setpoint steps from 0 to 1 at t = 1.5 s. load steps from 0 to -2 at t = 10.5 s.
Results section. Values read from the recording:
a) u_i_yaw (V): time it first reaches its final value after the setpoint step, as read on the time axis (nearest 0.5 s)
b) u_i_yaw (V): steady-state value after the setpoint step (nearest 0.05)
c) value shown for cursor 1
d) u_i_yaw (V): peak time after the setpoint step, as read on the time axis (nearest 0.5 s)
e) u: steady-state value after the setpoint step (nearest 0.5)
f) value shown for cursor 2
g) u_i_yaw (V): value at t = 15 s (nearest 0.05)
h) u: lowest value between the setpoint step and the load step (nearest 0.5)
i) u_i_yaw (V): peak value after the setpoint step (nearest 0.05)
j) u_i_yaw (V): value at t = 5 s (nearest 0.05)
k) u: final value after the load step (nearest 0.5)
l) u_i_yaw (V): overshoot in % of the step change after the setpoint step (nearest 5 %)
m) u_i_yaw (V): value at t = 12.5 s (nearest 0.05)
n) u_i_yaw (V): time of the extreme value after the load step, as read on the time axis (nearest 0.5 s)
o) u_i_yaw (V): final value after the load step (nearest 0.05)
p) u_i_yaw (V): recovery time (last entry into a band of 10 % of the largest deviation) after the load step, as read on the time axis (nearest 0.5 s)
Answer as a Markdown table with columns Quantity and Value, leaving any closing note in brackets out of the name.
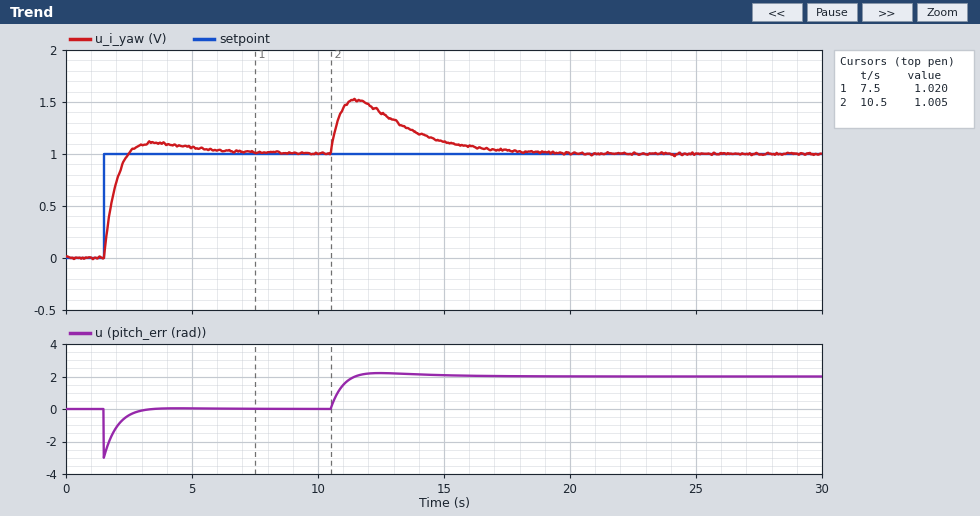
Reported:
| Quantity | Value |
|---|---|
| u_i_yaw (V): time it first reaches its final value after the setpoint step, as read on the time axis | 2.5 s |
| u_i_yaw (V): steady-state value after the setpoint step | 1.00 |
| value shown for cursor 1 | 1.020 |
| u_i_yaw (V): peak time after the setpoint step, as read on the time axis | 3.5 s |
| u: steady-state value after the setpoint step | 0.0 |
| value shown for cursor 2 | 1.005 |
| u_i_yaw (V): value at t = 15 s | 1.10 |
| u: lowest value between the setpoint step and the load step | -3.0 |
| u_i_yaw (V): peak value after the setpoint step | 1.10 |
| u_i_yaw (V): value at t = 5 s | 1.05 |
| u: final value after the load step | 2.0 |
| u_i_yaw (V): overshoot in % of the step change after the setpoint step | 10 % |
| u_i_yaw (V): value at t = 12.5 s | 1.40 |
| u_i_yaw (V): time of the extreme value after the load step, as read on the time axis | 11.5 s |
| u_i_yaw (V): final value after the load step | 1.00 |
| u_i_yaw (V): recovery time (last entry into a band of 10 % of the largest deviation) after the load step, as read on the time axis | 16.5 s |
